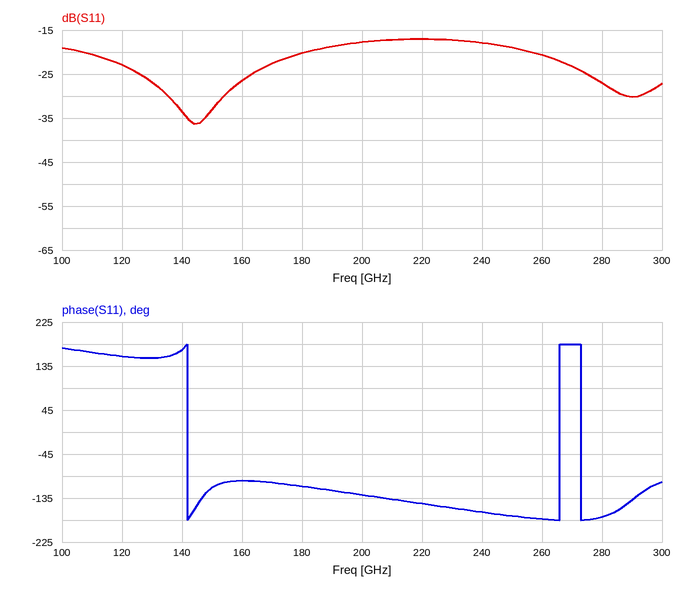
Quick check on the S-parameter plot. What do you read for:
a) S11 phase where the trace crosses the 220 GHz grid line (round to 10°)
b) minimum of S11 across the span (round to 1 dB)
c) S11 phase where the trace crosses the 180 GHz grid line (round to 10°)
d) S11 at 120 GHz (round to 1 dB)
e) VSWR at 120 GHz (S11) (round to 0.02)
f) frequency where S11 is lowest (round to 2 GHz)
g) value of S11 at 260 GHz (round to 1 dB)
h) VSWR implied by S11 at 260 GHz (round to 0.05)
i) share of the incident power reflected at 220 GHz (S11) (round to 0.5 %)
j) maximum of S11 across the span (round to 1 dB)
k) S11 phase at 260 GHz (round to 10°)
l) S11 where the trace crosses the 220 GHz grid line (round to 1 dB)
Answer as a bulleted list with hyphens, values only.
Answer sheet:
- -150°
- -36 dB
- -110°
- -23 dB
- 1.16
- 144 GHz
- -21 dB
- 1.20
- 2.0 %
- -17 dB
- -180°
- -17 dB
